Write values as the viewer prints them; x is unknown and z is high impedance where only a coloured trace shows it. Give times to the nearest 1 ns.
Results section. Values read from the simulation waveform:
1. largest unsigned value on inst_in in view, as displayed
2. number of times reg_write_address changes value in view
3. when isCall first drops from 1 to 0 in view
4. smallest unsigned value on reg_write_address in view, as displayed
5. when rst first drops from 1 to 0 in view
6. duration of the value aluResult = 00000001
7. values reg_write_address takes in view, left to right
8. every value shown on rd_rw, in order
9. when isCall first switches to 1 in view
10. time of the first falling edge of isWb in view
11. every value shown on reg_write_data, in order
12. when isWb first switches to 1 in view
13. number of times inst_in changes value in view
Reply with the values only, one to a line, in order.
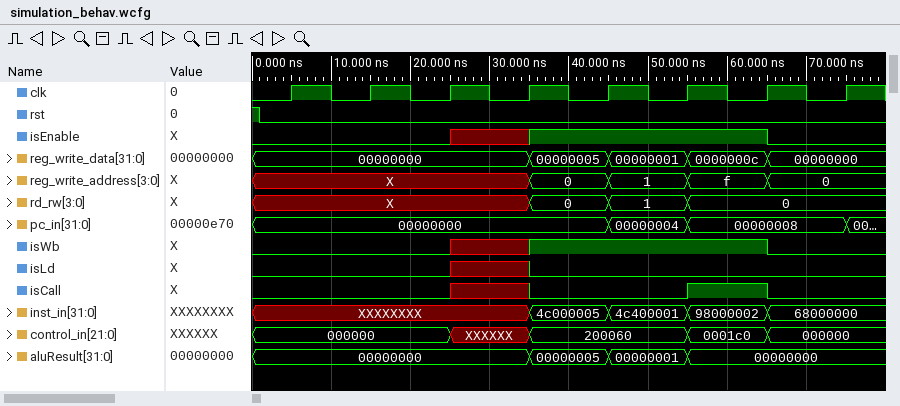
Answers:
98000002
4
65 ns
0
1 ns
10 ns
X, 0, 1, f, 0
X, 0, 1, 0
55 ns
65 ns
00000000, 00000005, 00000001, 0000000c, 00000000
35 ns
4
